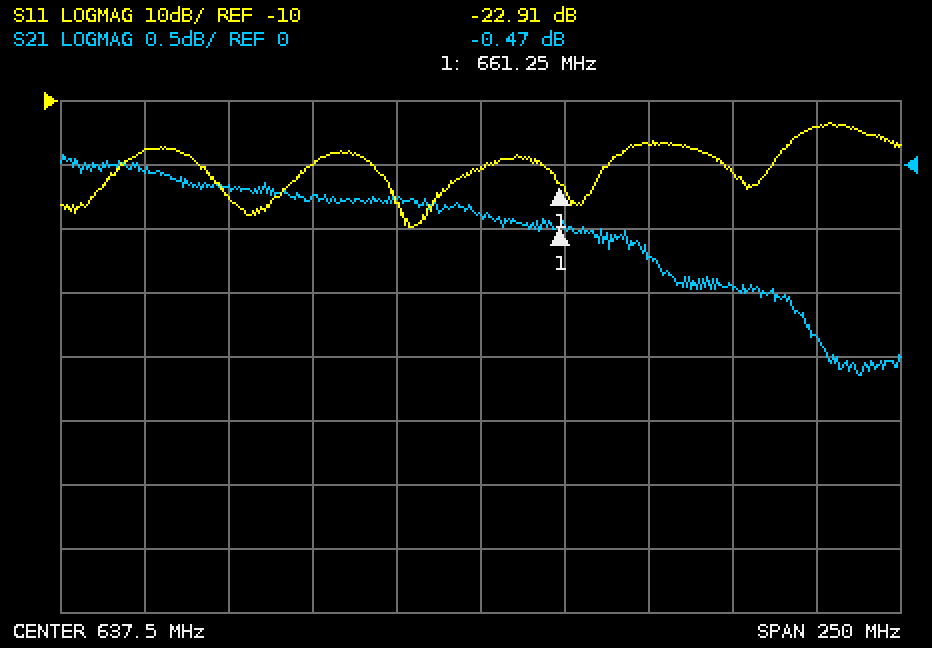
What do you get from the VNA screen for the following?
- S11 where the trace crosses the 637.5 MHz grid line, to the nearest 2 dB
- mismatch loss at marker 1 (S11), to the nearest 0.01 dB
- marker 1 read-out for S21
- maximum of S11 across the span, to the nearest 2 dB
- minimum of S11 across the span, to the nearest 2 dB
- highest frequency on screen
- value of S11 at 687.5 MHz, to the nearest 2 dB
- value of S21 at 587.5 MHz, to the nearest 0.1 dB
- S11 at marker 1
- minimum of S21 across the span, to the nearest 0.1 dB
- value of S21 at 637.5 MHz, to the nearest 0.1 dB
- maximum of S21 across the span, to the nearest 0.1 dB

-20 dB
0.02 dB
-0.47 dB
-14 dB
-30 dB
762.5 MHz
-16 dB
-0.2 dB
-22.91 dB
-1.6 dB
-0.4 dB
0.1 dB
